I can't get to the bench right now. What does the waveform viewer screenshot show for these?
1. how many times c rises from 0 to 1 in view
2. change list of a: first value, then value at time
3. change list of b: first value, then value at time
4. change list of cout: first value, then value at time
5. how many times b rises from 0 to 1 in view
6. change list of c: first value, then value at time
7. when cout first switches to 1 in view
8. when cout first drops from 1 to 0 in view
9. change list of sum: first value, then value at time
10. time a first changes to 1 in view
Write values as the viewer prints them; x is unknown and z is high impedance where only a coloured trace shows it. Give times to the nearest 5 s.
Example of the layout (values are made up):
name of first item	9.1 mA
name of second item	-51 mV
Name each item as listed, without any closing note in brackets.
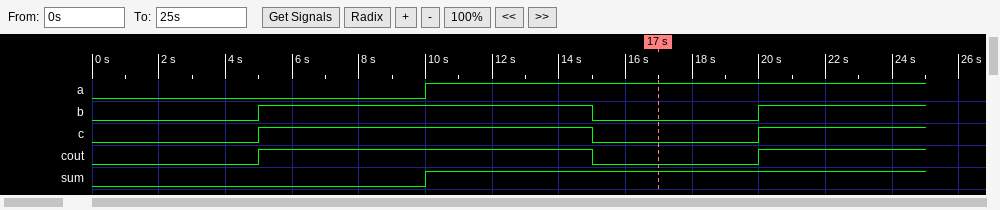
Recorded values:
how many times c rises from 0 to 1 in view	2
change list of a: first value, then value at time	0, 1 at 10 s
change list of b: first value, then value at time	0, 1 at 5 s, 0 at 15 s, 1 at 20 s
change list of cout: first value, then value at time	0, 1 at 5 s, 0 at 15 s, 1 at 20 s
how many times b rises from 0 to 1 in view	2
change list of c: first value, then value at time	0, 1 at 5 s, 0 at 15 s, 1 at 20 s
when cout first switches to 1 in view	5 s
when cout first drops from 1 to 0 in view	15 s
change list of sum: first value, then value at time	0, 1 at 10 s
time a first changes to 1 in view	10 s
